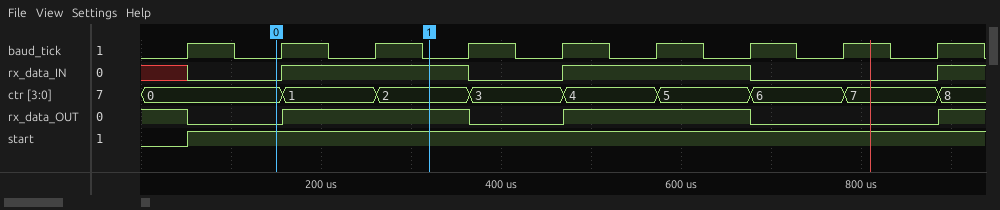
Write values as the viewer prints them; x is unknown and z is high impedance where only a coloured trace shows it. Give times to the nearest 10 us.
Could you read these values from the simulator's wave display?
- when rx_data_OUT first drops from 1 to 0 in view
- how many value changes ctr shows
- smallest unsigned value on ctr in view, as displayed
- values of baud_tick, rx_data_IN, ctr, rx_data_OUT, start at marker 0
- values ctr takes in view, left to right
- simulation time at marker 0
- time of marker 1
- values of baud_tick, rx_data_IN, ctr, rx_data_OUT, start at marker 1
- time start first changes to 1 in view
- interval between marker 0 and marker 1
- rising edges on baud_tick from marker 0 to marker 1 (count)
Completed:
50 us
8
0
baud_tick=0, rx_data_IN=0, ctr=0, rx_data_OUT=0, start=1
0, 1, 2, 3, 4, 5, 6, 7, 8
150 us
320 us
baud_tick=0, rx_data_IN=1, ctr=2, rx_data_OUT=1, start=1
50 us
170 us
2
